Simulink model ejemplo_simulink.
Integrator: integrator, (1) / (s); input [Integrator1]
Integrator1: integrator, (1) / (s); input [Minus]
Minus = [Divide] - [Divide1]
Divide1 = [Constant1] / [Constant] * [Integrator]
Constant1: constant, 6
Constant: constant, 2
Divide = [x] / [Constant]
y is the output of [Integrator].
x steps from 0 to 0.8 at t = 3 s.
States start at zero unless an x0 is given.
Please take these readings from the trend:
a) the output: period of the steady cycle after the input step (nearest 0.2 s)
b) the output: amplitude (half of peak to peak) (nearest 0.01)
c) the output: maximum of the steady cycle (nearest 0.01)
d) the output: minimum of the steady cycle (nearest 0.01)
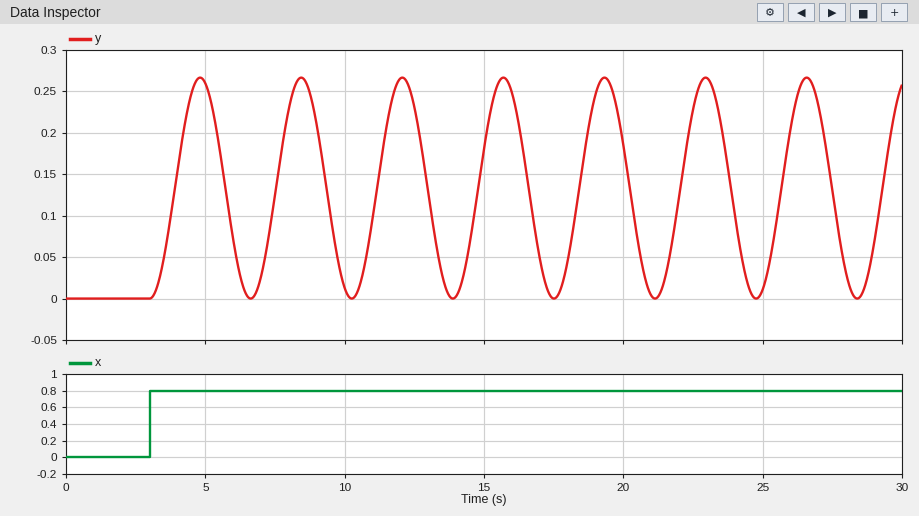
3.6 s
0.13
0.27
0.00
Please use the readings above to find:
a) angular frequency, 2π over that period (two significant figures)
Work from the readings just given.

1.7 rad/s
